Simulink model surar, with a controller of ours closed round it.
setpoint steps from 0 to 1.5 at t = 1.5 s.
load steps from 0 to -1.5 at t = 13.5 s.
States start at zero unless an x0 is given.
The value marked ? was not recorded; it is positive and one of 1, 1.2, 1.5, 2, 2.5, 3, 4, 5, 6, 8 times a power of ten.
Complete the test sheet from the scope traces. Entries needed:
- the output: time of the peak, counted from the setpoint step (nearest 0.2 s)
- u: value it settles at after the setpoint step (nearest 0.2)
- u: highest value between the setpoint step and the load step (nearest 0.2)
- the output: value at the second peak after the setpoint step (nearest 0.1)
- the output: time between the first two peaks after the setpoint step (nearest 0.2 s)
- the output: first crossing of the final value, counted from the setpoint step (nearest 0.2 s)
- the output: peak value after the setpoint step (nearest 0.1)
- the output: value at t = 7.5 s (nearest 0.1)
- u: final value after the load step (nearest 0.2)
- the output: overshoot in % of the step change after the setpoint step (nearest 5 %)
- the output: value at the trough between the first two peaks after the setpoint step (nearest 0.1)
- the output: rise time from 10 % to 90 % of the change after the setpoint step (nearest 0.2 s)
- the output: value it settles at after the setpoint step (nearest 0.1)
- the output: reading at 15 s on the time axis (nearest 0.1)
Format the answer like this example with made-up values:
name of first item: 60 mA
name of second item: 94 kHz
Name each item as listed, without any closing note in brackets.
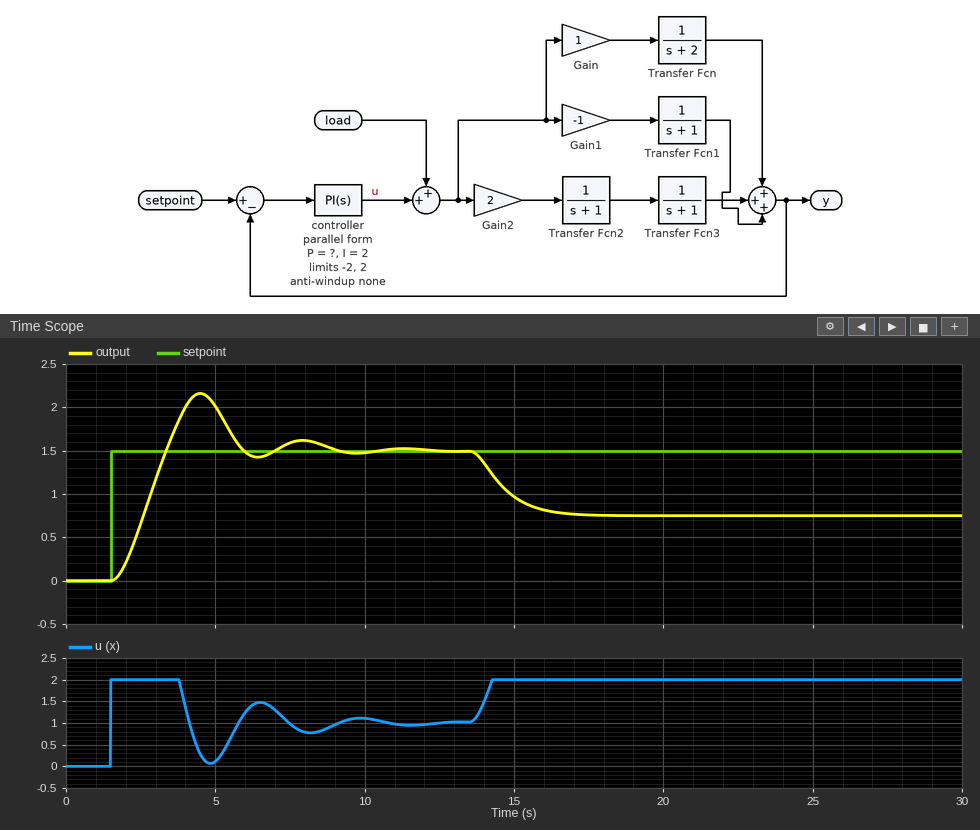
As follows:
the output: time of the peak, counted from the setpoint step: 3.0 s
u: value it settles at after the setpoint step: 1.0
u: highest value between the setpoint step and the load step: 2.0
the output: value at the second peak after the setpoint step: 1.6
the output: time between the first two peaks after the setpoint step: 3.4 s
the output: first crossing of the final value, counted from the setpoint step: 1.8 s
the output: peak value after the setpoint step: 2.2
the output: value at t = 7.5 s: 1.6
u: final value after the load step: 2.0
the output: overshoot in % of the step change after the setpoint step: 45 %
the output: value at the trough between the first two peaks after the setpoint step: 1.4
the output: rise time from 10 % to 90 % of the change after the setpoint step: 1.2 s
the output: value it settles at after the setpoint step: 1.5
the output: reading at 15 s on the time axis: 1.0
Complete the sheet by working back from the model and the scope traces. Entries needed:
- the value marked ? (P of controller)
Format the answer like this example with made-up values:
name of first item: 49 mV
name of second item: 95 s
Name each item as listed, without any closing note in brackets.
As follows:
the value marked ?: 3
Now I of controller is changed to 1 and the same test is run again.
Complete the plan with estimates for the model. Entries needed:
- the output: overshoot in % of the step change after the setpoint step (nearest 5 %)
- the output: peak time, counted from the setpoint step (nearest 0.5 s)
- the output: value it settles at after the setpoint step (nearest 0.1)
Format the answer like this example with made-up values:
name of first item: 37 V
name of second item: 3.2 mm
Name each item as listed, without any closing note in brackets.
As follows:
the output: overshoot in % of the step change after the setpoint step: 25 %
the output: peak time, counted from the setpoint step: 2.5 s
the output: value it settles at after the setpoint step: 1.5
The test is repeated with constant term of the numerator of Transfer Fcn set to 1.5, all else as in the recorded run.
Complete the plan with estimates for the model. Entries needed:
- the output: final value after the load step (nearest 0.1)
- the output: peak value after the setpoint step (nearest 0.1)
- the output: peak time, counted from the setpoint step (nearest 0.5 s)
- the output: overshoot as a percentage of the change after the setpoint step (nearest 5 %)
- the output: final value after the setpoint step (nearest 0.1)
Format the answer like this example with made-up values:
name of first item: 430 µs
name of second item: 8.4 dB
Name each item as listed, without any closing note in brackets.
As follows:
the output: final value after the load step: 0.9
the output: peak value after the setpoint step: 1.9
the output: peak time, counted from the setpoint step: 2.0 s
the output: overshoot as a percentage of the change after the setpoint step: 25 %
the output: final value after the setpoint step: 1.5
